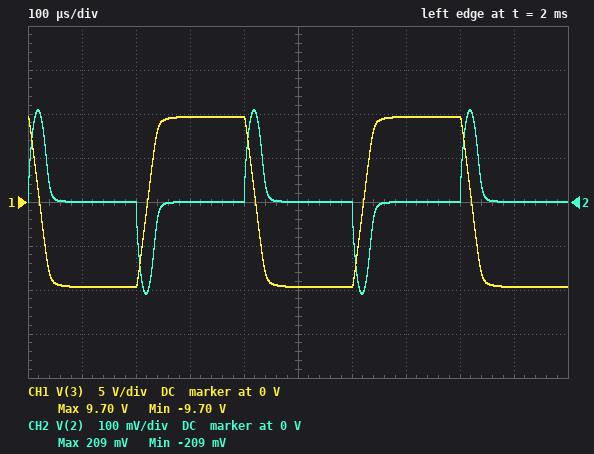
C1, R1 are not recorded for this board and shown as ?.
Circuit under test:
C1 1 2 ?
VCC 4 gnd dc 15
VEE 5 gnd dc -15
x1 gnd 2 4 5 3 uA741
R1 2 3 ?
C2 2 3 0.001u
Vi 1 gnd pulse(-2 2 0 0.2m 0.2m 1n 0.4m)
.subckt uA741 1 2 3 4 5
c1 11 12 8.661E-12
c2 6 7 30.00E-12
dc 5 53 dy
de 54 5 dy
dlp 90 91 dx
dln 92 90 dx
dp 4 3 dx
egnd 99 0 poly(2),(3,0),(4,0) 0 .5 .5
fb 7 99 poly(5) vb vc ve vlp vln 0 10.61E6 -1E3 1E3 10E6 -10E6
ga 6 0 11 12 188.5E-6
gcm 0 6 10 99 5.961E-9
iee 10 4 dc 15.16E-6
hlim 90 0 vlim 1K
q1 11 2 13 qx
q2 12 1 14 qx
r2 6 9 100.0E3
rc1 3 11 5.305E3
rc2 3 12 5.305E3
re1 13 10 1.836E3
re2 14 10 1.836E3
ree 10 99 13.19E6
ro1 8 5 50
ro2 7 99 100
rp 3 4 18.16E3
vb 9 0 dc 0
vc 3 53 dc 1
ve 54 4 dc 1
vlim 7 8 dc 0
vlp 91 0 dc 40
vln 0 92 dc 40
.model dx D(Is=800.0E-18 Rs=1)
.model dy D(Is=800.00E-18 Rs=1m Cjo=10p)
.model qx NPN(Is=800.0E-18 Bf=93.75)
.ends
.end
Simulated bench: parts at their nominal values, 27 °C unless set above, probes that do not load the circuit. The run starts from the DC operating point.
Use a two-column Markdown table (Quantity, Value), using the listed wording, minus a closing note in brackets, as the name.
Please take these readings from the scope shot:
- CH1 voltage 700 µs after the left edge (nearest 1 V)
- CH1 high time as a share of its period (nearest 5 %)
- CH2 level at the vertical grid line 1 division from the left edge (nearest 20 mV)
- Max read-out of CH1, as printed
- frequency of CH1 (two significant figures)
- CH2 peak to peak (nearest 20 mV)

| Quantity | Value |
|---|---|
| CH1 voltage 700 µs after the left edge | 10 V |
| CH1 high time as a share of its period | 50 % |
| CH2 level at the vertical grid line 1 division from the left edge | 0 V |
| Max read-out of CH1, as printed | 9.70 V |
| frequency of CH1 | 2.5 kHz |
| CH2 peak to peak | 420 mV |
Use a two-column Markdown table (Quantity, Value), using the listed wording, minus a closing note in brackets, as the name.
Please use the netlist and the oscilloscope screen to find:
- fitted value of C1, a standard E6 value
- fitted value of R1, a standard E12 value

| Quantity | Value |
|---|---|
| fitted value of C1, a standard E6 value | 22 nF |
| fitted value of R1, a standard E12 value | 22 kΩ |
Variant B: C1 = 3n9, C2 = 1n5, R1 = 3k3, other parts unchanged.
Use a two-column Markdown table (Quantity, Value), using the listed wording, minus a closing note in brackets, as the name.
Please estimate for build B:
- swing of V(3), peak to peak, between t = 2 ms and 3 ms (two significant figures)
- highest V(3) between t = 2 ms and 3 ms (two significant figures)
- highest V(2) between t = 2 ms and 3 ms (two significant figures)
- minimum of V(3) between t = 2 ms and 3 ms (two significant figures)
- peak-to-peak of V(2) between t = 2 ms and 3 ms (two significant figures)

| Quantity | Value |
|---|---|
| swing of V(3), peak to peak, between t = 2 ms and 3 ms | 520 mV |
| highest V(3) between t = 2 ms and 3 ms | 260 mV |
| highest V(2) between t = 2 ms and 3 ms | 15 mV |
| minimum of V(3) between t = 2 ms and 3 ms | -260 mV |
| peak-to-peak of V(2) between t = 2 ms and 3 ms | 29 mV |
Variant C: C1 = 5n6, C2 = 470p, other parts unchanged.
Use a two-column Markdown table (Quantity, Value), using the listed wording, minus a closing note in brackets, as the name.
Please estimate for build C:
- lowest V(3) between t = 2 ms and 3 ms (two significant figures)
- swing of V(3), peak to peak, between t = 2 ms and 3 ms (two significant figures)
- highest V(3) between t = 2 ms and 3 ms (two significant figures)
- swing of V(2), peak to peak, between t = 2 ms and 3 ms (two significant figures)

| Quantity | Value |
|---|---|
| lowest V(3) between t = 2 ms and 3 ms | -2.5 V |
| swing of V(3), peak to peak, between t = 2 ms and 3 ms | 4.9 V |
| highest V(3) between t = 2 ms and 3 ms | 2.5 V |
| swing of V(2), peak to peak, between t = 2 ms and 3 ms | 130 mV |
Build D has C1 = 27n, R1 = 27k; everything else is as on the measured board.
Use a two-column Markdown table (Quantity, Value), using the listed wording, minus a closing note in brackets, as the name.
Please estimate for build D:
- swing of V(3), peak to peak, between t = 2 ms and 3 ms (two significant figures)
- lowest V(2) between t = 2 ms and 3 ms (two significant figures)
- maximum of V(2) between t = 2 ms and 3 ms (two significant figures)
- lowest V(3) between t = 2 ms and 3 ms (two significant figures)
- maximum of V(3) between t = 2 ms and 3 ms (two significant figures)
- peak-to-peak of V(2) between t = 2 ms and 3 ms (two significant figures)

| Quantity | Value |
|---|---|
| swing of V(3), peak to peak, between t = 2 ms and 3 ms | 30 V |
| lowest V(2) between t = 2 ms and 3 ms | -560 mV |
| maximum of V(2) between t = 2 ms and 3 ms | 560 mV |
| lowest V(3) between t = 2 ms and 3 ms | -15 V |
| maximum of V(3) between t = 2 ms and 3 ms | 15 V |
| peak-to-peak of V(2) between t = 2 ms and 3 ms | 1.1 V |
